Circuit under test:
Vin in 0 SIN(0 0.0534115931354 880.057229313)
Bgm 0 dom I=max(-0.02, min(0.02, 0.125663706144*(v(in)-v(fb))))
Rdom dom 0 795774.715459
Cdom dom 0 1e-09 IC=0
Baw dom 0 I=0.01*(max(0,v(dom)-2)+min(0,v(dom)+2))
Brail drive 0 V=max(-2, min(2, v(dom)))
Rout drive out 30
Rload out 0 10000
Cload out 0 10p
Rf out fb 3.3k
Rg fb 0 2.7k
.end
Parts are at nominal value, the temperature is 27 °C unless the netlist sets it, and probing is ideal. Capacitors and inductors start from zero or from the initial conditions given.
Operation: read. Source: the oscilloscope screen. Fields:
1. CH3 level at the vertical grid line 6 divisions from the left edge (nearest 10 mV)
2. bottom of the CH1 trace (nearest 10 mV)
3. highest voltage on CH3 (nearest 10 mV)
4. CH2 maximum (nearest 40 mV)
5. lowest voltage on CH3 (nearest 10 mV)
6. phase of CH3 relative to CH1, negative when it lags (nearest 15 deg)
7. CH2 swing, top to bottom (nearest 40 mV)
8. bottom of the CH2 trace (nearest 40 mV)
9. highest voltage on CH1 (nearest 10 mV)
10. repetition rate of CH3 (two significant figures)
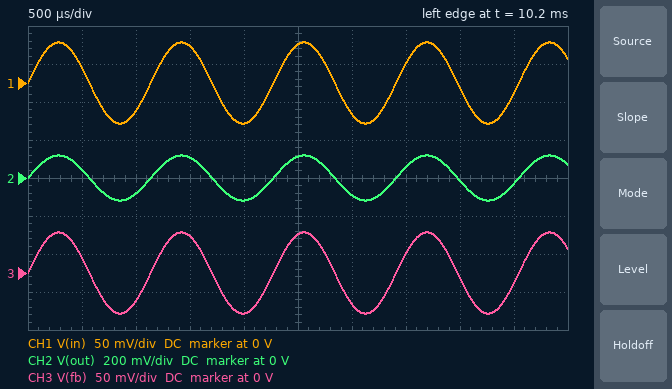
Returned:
-40 mV
-50 mV
50 mV
120 mV
-50 mV
0 deg
240 mV
-120 mV
50 mV
880 Hz
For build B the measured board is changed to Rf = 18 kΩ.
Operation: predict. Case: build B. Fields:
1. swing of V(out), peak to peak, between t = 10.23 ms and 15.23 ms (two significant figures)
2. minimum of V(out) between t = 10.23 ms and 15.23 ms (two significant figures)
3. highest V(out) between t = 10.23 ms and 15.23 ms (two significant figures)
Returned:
820 mV
-410 mV
410 mV
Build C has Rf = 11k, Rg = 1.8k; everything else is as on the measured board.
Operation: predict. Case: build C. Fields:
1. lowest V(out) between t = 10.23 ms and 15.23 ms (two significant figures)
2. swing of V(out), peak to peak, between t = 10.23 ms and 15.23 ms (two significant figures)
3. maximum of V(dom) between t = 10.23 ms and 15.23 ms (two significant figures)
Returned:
-380 mV
760 mV
380 mV
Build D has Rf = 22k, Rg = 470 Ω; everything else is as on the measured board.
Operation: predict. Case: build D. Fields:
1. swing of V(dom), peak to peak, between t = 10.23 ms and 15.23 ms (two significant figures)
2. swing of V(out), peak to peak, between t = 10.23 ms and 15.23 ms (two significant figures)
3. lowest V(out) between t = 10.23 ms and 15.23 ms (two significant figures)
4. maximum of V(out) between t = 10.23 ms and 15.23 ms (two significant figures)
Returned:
4.3 V
4.0 V
-2.0 V
2.0 V
